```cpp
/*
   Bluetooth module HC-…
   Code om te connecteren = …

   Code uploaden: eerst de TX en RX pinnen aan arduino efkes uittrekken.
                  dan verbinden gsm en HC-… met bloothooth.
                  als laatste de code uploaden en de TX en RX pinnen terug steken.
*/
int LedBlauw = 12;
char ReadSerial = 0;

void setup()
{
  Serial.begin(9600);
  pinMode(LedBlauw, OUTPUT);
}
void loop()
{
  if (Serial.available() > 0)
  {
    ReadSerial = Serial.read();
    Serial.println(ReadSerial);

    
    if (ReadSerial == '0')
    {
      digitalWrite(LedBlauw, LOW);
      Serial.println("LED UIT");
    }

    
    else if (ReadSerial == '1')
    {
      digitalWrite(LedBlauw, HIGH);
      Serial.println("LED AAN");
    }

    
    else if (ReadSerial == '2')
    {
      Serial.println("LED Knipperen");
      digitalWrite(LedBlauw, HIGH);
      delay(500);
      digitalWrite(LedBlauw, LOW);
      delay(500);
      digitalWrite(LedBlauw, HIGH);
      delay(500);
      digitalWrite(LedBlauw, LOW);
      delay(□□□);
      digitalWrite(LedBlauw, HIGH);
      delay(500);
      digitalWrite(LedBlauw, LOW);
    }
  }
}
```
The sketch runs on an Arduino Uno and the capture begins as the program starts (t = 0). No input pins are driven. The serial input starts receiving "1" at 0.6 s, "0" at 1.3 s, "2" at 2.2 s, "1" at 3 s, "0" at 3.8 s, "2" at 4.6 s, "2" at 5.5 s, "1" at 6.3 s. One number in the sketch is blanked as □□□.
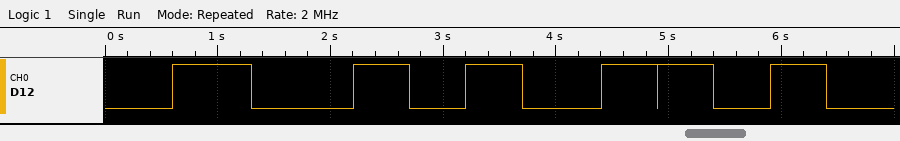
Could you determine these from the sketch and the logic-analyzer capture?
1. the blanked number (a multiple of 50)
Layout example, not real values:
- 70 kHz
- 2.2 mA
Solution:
- 700
